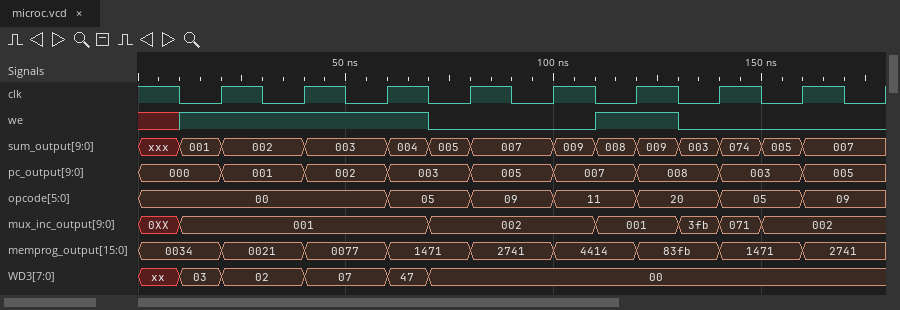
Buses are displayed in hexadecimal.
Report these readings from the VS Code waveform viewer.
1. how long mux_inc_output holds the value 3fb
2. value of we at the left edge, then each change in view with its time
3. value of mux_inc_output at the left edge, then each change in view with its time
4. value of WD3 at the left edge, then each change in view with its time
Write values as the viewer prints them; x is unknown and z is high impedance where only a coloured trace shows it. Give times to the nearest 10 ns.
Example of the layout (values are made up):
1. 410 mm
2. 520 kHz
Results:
1. 10 ns
2. x, 1 at 10 ns, 0 at 70 ns, 1 at 110 ns, 0 at 130 ns
3. 0XX, 001 at 10 ns, 002 at 70 ns, 001 at 110 ns, 3fb at 130 ns, 071 at 140 ns, 002 at 150 ns
4. xx, 03 at 10 ns, 02 at 20 ns, 07 at 40 ns, 47 at 60 ns, 00 at 70 ns
